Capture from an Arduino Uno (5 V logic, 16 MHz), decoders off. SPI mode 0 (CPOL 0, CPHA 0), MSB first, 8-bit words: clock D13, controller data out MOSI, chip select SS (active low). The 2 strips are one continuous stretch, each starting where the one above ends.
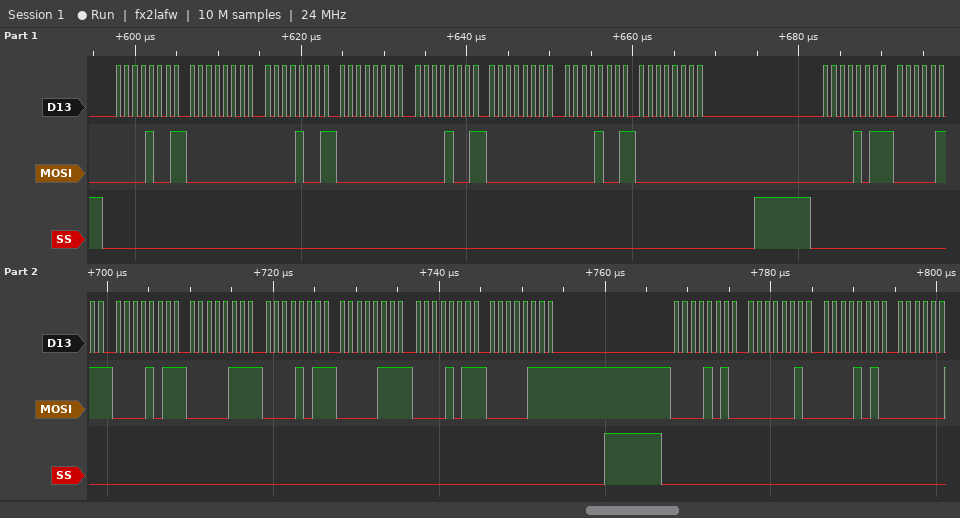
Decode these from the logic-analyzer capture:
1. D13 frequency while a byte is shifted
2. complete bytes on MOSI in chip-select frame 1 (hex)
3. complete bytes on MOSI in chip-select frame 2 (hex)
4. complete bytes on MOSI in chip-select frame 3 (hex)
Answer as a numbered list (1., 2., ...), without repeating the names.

1. 1 MHz
2. 09 00 09 00 09 00 09 00
3. 0B 07 0B 07 0B 07 0B 07
4. 0A 02 0A
